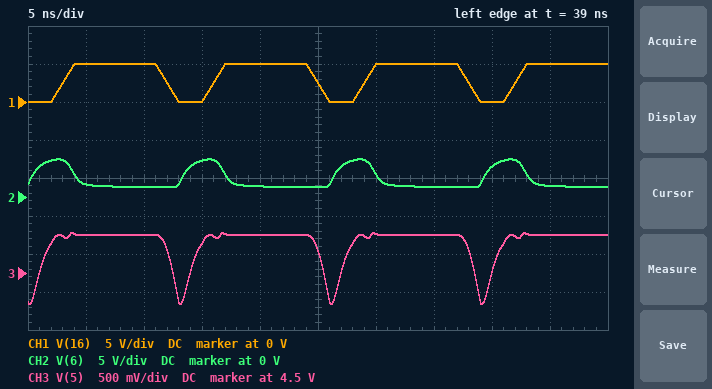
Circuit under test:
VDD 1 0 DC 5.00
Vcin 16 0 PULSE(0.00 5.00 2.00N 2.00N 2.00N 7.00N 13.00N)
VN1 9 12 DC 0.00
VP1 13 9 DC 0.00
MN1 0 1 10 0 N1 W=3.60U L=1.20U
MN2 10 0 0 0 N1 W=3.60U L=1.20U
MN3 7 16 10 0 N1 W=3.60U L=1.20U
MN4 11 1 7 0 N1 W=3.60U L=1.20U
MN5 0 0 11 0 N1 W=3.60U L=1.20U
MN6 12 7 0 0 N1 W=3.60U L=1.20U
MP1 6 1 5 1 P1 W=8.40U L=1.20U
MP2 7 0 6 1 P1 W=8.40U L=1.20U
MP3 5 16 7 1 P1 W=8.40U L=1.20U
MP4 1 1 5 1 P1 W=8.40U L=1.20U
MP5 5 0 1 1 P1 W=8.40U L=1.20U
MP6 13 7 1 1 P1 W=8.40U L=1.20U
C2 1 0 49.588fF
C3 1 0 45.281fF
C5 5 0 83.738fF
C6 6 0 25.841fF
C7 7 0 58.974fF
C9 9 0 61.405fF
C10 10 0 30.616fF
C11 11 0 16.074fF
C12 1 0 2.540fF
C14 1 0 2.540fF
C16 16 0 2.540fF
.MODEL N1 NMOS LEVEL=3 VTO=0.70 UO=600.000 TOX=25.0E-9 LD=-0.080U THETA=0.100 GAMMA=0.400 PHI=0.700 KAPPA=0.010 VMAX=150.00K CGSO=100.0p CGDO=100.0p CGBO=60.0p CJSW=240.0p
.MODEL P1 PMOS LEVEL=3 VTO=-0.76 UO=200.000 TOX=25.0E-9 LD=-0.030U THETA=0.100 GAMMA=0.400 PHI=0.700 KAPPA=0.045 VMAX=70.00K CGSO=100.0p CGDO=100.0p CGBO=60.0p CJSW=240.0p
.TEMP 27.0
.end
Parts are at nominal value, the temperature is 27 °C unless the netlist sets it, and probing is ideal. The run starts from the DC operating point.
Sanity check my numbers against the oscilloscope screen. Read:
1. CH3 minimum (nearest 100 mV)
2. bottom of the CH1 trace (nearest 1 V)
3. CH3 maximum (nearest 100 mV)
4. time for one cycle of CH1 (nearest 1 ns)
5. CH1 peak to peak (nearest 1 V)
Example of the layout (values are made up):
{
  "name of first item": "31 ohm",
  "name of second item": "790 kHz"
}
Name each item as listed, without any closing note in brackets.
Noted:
{
  "CH3 minimum": "4.1 V",
  "bottom of the CH1 trace": "0 V",
  "CH3 maximum": "5.0 V",
  "time for one cycle of CH1": "13 ns",
  "CH1 peak to peak": "5 V"
}
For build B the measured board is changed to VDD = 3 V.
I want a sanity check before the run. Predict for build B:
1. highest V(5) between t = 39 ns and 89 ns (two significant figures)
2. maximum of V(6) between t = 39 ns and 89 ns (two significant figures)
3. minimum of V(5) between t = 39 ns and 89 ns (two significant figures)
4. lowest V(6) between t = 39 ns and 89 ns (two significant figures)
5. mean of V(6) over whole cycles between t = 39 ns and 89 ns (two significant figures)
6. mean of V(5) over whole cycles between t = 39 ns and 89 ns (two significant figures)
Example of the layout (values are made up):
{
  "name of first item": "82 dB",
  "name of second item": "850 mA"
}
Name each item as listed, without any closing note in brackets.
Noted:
{
  "highest V(5) between t = 39 ns and 89 ns": "3.0 V",
  "maximum of V(6) between t = 39 ns and 89 ns": "2.6 V",
  "minimum of V(5) between t = 39 ns and 89 ns": "2.5 V",
  "lowest V(6) between t = 39 ns and 89 ns": "1.1 V",
  "mean of V(6) over whole cycles between t = 39 ns and 89 ns": "1.4 V",
  "mean of V(5) over whole cycles between t = 39 ns and 89 ns": "2.9 V"
}
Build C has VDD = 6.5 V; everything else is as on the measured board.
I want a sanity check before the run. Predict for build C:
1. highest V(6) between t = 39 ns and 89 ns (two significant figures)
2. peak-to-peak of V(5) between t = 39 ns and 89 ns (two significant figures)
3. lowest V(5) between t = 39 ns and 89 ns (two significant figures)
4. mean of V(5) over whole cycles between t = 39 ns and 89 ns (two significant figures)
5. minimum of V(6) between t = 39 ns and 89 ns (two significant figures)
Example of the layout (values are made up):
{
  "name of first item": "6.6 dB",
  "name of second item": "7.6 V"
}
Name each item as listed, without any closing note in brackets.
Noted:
{
  "highest V(6) between t = 39 ns and 89 ns": "6.5 V",
  "peak-to-peak of V(5) between t = 39 ns and 89 ns": "1.1 V",
  "lowest V(5) between t = 39 ns and 89 ns": "5.4 V",
  "mean of V(5) over whole cycles between t = 39 ns and 89 ns": "6.3 V",
  "minimum of V(6) between t = 39 ns and 89 ns": "1.4 V"
}
